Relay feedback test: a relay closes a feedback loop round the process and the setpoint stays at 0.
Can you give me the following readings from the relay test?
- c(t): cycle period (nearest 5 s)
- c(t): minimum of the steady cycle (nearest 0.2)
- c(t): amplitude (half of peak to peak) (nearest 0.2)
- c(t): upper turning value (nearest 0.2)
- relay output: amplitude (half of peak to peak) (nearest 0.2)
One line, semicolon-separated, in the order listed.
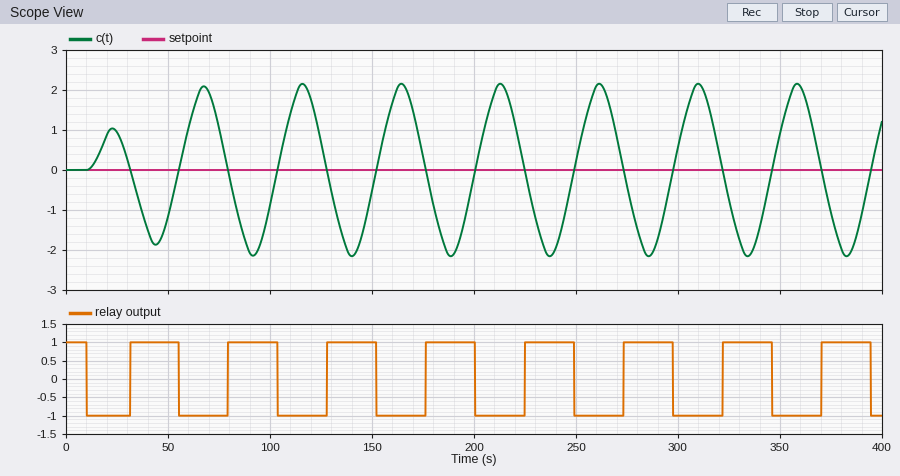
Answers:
50 s; -2.2; 2.2; 2.2; 1.0
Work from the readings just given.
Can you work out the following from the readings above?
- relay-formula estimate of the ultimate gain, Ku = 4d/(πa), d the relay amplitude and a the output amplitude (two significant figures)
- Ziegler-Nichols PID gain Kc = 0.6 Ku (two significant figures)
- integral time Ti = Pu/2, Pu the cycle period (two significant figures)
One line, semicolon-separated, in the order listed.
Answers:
0.58; 0.35; 25 s
